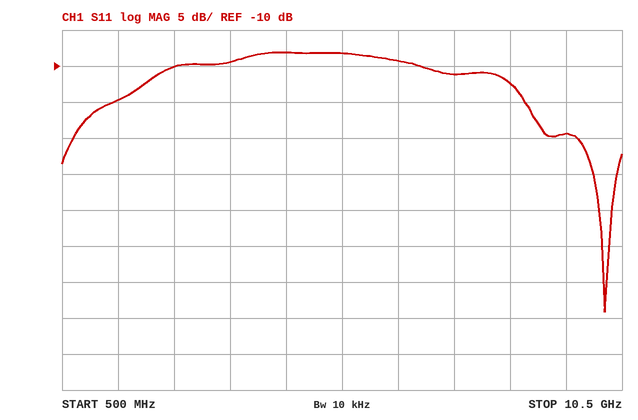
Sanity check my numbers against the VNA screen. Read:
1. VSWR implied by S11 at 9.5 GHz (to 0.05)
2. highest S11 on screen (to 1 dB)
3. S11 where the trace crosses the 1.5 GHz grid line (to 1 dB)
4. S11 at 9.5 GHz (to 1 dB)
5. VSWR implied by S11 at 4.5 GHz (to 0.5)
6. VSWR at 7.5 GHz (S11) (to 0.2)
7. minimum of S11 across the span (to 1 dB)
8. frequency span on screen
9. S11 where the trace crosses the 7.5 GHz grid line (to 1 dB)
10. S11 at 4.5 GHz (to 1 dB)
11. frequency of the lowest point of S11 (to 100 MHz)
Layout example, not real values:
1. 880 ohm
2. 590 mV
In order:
1. 1.25
2. -8 dB
3. -15 dB
4. -19 dB
5. 2.5
6. 1.8
7. -44 dB
8. 10 GHz
9. -11 dB
10. -8 dB
11. 10.2 GHz
